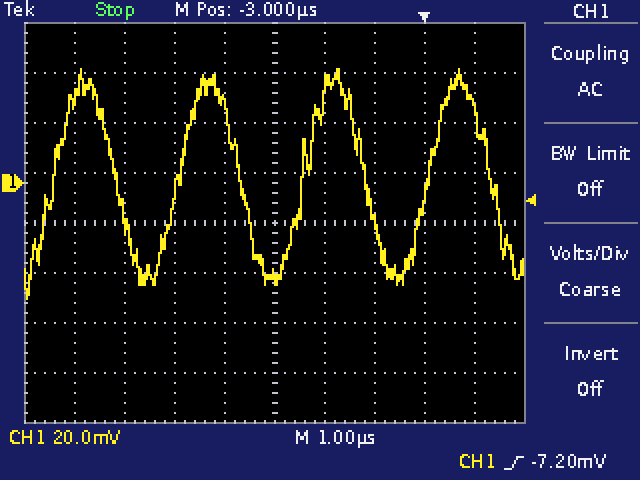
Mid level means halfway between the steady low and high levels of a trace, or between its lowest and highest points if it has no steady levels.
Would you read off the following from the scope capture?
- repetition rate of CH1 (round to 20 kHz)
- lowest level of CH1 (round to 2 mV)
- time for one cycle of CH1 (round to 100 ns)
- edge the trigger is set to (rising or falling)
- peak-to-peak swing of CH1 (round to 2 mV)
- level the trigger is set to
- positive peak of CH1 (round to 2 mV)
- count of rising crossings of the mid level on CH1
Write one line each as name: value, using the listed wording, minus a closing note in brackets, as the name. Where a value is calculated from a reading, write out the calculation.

repetition rate of CH1: 1 / 2.5 µs ≈ 400 kHz
lowest level of CH1: -46 mV
time for one cycle of CH1: 2.5 µs
edge the trigger is set to: rising
peak-to-peak swing of CH1: 46 mV − (-46 mV) = 92 mV
level the trigger is set to: -7.20 mV
positive peak of CH1: 46 mV
count of rising crossings of the mid level on CH1: 4
